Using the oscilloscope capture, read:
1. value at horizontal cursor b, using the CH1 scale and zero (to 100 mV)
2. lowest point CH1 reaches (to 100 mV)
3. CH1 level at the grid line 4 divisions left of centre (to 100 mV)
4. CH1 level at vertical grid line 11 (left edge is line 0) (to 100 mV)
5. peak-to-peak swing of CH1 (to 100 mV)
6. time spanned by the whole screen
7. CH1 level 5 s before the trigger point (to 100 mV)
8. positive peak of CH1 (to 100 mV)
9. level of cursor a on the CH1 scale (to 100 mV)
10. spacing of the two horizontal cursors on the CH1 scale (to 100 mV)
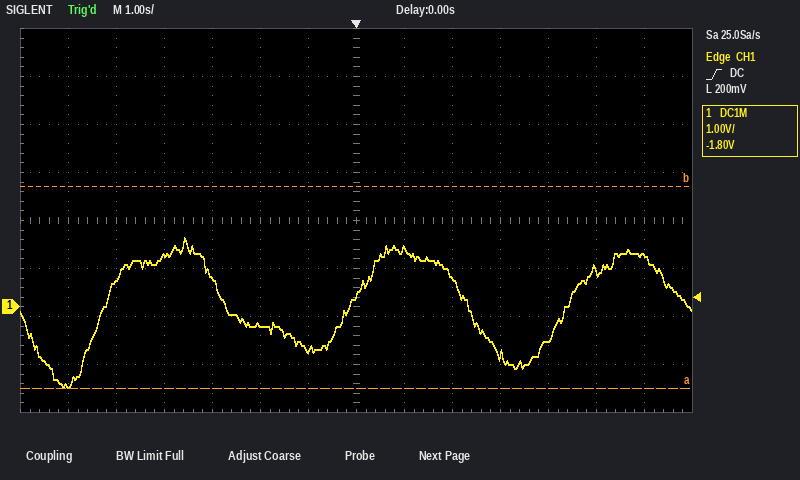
2.5 V
-1.7 V
1.1 V
-700 mV
3.1 V
14 s
500 mV
1.4 V
-1.7 V
4.2 V
